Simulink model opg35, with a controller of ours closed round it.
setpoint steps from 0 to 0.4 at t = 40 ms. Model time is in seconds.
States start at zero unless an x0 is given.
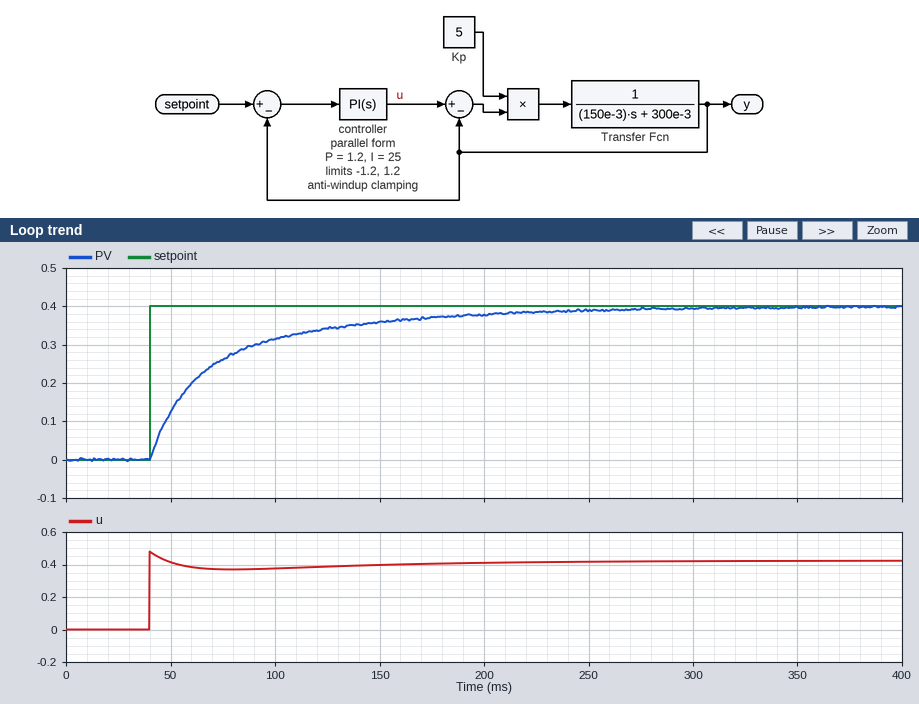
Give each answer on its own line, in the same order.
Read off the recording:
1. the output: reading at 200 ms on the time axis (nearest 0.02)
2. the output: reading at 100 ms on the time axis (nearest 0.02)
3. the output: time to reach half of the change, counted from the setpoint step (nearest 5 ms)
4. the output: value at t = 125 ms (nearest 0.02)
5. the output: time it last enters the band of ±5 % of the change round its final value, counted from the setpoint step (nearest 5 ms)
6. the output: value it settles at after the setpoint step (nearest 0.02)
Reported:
0.38
0.32
20 ms
0.34
165 ms
0.40
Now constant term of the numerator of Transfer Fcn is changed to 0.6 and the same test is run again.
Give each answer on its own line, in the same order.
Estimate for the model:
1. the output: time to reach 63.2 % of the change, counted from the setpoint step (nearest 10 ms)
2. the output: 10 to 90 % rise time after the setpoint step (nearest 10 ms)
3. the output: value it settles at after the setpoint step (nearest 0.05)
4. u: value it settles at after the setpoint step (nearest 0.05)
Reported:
40 ms
100 ms
0.40
0.45
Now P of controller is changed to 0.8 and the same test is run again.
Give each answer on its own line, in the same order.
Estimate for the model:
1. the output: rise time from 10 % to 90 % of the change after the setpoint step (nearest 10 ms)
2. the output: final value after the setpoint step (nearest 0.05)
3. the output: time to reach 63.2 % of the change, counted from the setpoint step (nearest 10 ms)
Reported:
100 ms
0.40
40 ms
